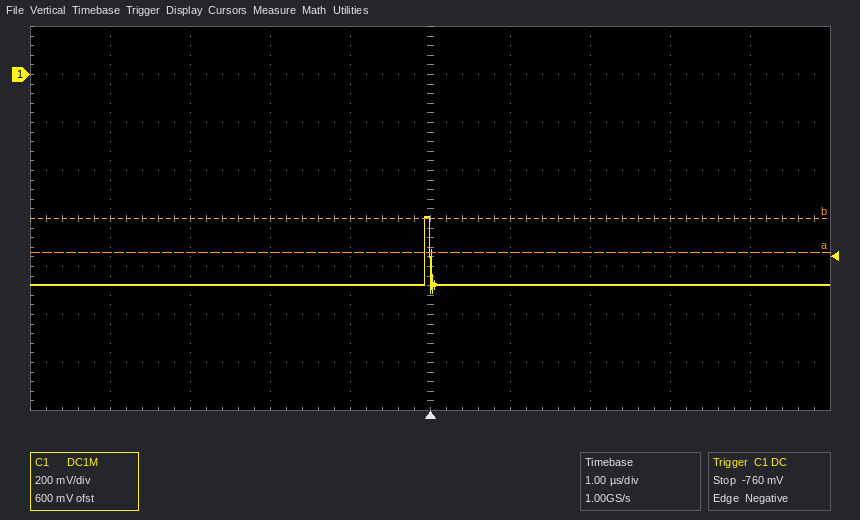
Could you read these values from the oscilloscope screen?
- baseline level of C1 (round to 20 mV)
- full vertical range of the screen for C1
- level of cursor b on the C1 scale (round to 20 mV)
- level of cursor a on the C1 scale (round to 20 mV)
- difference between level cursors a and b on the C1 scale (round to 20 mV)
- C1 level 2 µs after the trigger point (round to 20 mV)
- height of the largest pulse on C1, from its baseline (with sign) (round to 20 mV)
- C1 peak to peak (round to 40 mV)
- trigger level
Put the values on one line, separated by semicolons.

-880 mV; 1.6 V; -600 mV; -740 mV; 140 mV; -880 mV; +280 mV; 320 mV; -760 mV
